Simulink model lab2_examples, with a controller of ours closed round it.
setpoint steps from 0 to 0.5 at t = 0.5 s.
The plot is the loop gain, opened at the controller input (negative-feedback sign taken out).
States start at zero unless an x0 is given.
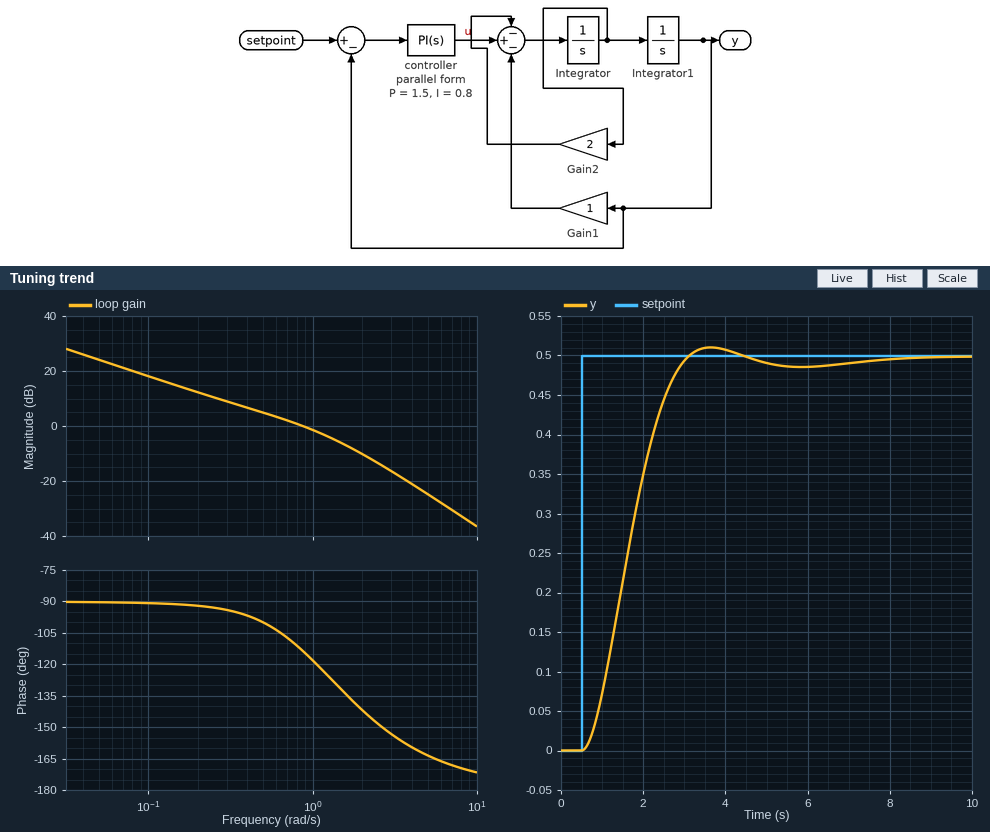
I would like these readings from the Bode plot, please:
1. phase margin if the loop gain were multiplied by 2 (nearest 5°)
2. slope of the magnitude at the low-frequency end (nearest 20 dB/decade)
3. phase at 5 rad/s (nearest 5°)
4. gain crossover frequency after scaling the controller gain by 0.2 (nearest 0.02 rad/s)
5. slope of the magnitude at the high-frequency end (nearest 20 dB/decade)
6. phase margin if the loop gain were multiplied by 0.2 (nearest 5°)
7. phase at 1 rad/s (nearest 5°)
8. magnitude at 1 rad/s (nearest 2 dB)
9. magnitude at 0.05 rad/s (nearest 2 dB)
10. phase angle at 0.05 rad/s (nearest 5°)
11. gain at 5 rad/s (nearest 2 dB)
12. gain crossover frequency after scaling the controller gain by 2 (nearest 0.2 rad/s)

50°
-20 dB/decade
-165°
0.16 rad/s
-40 dB/decade
90°
-120°
-2 dB
24 dB
-90°
-24 dB
1.4 rad/s
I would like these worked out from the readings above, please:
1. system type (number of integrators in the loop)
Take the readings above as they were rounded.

1
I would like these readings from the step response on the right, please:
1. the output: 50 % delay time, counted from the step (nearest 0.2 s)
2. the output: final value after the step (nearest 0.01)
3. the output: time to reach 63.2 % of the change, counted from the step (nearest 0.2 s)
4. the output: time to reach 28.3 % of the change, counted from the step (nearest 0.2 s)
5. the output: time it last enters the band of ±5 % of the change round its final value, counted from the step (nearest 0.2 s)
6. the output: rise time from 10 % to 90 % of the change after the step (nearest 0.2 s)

1.2 s
0.50
1.4 s
0.8 s
2.2 s
1.6 s
